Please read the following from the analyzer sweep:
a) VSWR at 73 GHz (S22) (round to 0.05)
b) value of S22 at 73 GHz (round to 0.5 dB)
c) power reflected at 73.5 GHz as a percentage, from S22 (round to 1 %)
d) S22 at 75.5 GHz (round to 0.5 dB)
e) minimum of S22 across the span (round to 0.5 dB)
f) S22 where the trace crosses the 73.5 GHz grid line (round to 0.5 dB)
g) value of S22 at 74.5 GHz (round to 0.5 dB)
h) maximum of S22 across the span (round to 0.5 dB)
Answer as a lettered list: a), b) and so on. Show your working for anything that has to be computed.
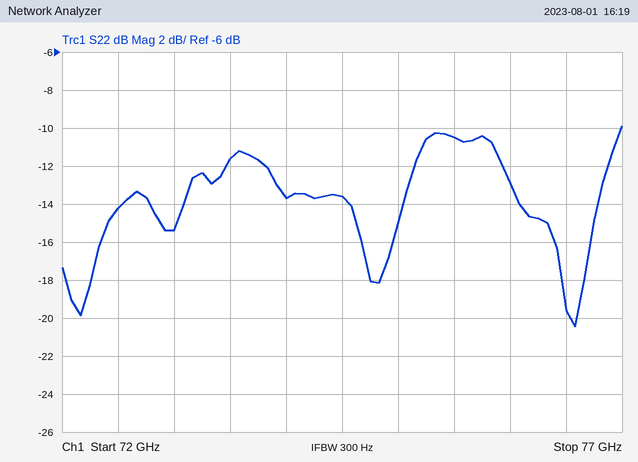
a) |Γ| = 10^(-15.5/20) = 0.1679; VSWR = (1 + 0.1679)/(1 − 0.1679) ≈ 1.40
b) -15.5 dB
c) 10^(-11.5/10) ≈ 7 %
d) -10.5 dB
e) -20.5 dB
f) -11.5 dB
g) -13.5 dB
h) -10.0 dB
